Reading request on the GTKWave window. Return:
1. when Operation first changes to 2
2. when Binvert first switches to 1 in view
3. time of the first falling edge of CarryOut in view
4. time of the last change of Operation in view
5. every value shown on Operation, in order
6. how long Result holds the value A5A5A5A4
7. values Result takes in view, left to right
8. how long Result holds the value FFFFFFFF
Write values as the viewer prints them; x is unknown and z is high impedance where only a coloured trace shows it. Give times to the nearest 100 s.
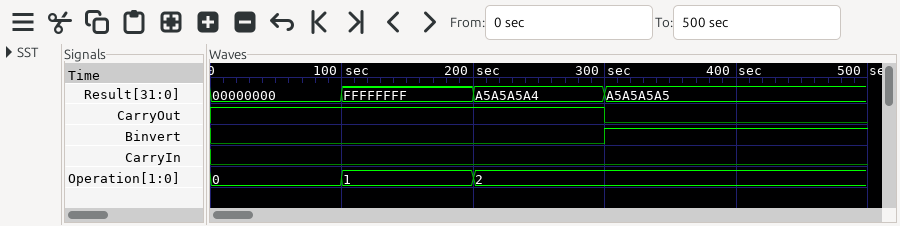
200 s
300 s
300 s
200 s
0, 1, 2
100 s
00000000, FFFFFFFF, A5A5A5A4, A5A5A5A5
100 s
